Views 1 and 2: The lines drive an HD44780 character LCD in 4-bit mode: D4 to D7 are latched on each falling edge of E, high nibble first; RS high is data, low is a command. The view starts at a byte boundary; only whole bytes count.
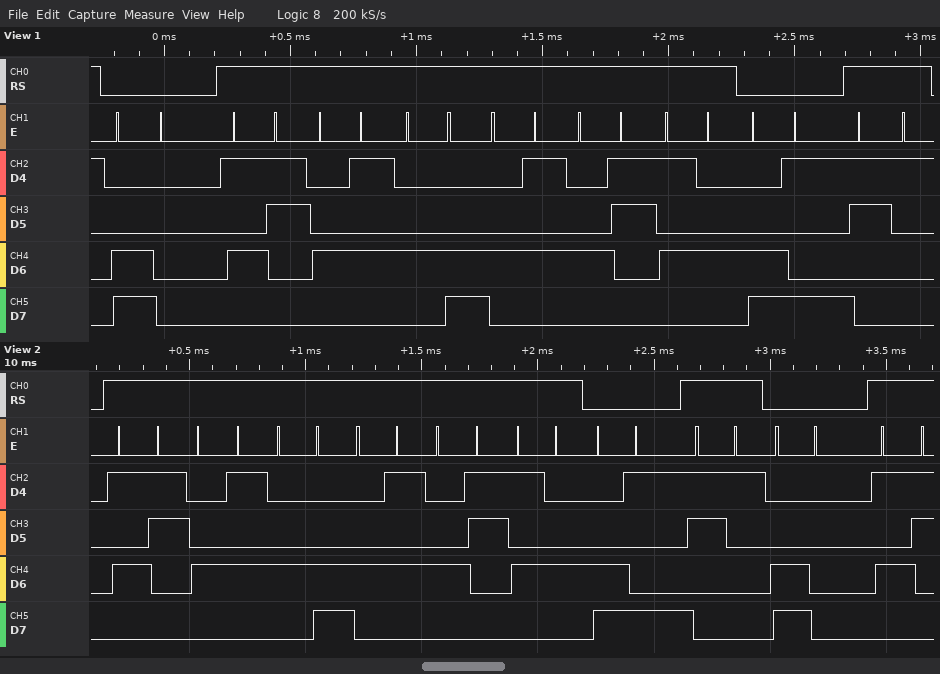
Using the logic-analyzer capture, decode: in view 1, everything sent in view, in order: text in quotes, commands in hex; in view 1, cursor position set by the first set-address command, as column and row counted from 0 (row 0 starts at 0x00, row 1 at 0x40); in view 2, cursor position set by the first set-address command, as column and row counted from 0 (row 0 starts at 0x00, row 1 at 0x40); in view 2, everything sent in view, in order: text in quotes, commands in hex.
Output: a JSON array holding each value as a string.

["0xC0 \"SELECT\" 0xC9 \"1\"", "column 0, row 1", "column 9, row 1", "\"SELECT\" 0xC9 \"1\" 0xC0 \"S\""]
